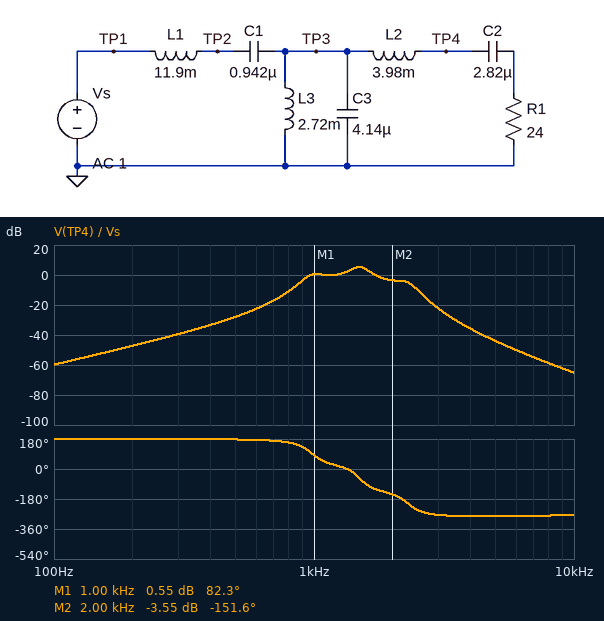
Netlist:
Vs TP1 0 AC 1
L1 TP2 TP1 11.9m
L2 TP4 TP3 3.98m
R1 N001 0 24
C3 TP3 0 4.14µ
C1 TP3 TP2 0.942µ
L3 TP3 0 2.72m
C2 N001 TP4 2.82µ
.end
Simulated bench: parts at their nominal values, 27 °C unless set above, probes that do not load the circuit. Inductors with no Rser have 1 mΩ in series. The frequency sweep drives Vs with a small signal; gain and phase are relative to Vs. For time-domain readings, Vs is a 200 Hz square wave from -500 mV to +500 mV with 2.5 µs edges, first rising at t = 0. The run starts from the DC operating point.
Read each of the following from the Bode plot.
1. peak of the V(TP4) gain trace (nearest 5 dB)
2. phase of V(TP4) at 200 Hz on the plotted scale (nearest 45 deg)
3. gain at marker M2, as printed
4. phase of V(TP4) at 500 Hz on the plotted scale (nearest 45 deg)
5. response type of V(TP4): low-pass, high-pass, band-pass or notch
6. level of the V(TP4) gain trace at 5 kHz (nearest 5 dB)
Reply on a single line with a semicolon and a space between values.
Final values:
5 dB; 180 deg; -3.55 dB; 180 deg; band-pass; -45 dB
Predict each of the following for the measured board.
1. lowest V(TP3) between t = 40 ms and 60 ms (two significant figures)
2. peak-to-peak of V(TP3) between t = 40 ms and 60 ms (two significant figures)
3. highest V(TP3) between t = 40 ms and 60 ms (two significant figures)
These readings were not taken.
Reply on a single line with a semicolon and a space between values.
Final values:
-270 mV; 540 mV; 270 mV
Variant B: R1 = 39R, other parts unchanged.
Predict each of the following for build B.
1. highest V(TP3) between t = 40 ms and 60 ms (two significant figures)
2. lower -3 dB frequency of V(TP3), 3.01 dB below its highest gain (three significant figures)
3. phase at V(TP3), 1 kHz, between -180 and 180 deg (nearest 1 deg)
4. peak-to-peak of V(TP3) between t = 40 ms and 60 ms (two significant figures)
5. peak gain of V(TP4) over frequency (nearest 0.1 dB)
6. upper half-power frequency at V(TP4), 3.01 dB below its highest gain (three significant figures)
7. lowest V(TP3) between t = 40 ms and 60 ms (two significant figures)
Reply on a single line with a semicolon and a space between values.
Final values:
280 mV; 1.06 kHz; 121 deg; 550 mV; 2.9 dB; 1.83 kHz; -280 mV
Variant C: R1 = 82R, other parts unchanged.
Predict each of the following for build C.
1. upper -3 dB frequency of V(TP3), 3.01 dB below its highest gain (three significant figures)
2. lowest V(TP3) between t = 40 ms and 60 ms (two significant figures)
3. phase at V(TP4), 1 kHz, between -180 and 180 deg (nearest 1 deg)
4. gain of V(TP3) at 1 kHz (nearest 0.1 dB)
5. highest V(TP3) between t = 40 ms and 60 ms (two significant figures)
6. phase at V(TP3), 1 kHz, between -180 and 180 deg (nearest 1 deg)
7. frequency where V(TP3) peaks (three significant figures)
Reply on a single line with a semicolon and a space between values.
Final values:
2.03 kHz; -290 mV; 136 deg; -5.8 dB; 290 mV; 149 deg; 1.88 kHz
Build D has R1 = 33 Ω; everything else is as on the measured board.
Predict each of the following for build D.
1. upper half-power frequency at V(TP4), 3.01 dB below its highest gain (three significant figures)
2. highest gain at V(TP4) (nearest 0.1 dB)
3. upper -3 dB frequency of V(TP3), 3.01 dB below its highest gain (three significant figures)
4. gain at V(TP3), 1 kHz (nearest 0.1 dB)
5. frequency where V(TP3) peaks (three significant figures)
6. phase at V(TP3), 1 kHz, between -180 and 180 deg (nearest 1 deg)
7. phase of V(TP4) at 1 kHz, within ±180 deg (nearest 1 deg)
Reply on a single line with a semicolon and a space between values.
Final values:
1.72 kHz; 3.6 dB; 1.88 kHz; -4.2 dB; 1.50 kHz; 113 deg; 97 deg
